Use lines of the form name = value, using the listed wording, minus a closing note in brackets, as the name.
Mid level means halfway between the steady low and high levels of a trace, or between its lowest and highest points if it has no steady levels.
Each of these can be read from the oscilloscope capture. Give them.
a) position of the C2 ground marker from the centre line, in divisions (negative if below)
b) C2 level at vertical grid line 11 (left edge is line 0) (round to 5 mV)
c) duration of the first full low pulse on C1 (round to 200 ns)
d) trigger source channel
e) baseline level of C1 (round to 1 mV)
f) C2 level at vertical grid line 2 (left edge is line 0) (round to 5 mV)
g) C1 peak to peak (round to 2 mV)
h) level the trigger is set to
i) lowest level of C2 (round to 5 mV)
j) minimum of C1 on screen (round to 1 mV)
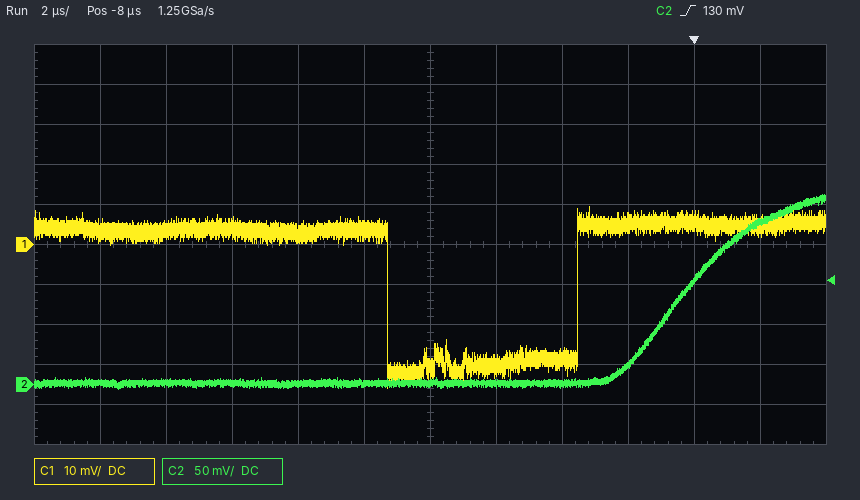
position of the C2 ground marker from the centre line, in divisions = -3.5 div
C2 level at vertical grid line 11 (left edge is line 0) = 205 mV
duration of the first full low pulse on C1 = 5.8 µs
trigger source channel = C2
baseline level of C1 = 4 mV
C2 level at vertical grid line 2 (left edge is line 0) = 0 mV
C1 peak to peak = 46 mV
level the trigger is set to = 130 mV
lowest level of C2 = -5 mV
minimum of C1 on screen = -36 mV
